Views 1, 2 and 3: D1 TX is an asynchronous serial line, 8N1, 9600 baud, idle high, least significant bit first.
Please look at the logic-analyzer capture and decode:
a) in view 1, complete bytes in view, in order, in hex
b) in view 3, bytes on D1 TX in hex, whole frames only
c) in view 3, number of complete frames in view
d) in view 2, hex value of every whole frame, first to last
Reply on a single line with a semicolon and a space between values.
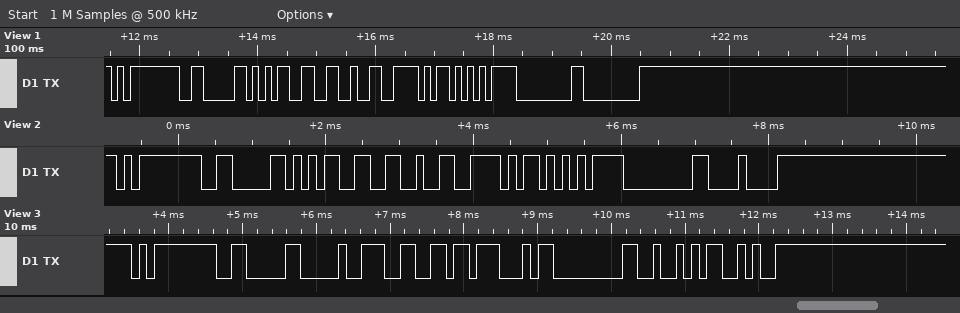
FD 06 35 26 5E D5 00 00; FD 06 90 66 47 00 52 CA; 8; FD 06 35 26 5E D5 00 08
